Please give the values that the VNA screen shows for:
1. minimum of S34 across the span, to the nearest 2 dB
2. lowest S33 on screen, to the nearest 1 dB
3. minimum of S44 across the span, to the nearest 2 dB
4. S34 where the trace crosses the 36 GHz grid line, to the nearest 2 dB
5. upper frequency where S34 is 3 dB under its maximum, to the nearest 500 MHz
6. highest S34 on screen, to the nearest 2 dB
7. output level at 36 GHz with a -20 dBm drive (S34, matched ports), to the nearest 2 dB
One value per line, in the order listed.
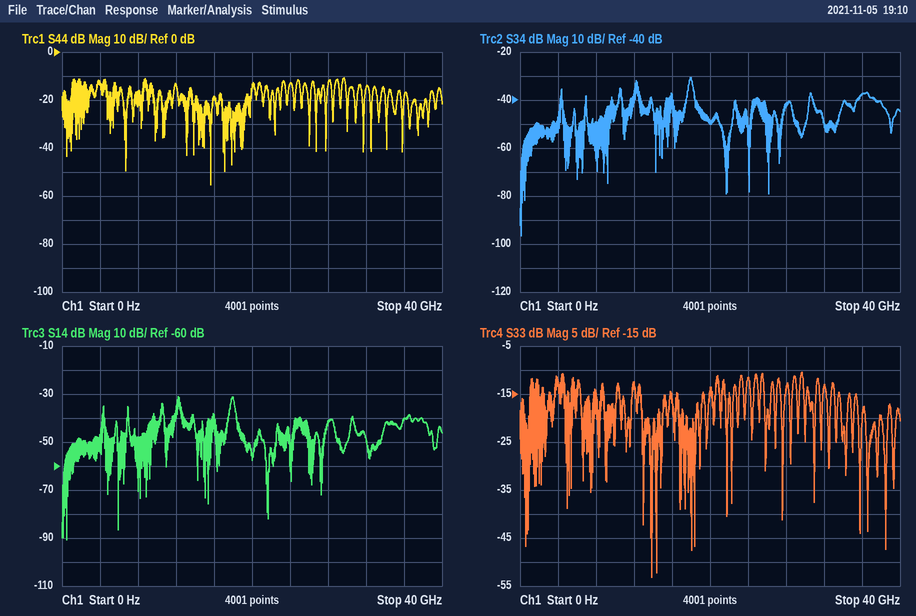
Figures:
-96 dB
-53 dB
-56 dB
-38 dB
18.0 GHz
-30 dB
-58 dBm
